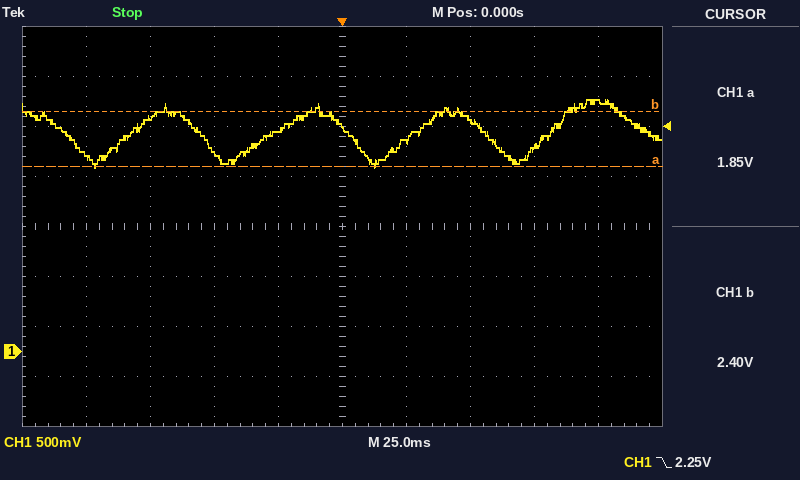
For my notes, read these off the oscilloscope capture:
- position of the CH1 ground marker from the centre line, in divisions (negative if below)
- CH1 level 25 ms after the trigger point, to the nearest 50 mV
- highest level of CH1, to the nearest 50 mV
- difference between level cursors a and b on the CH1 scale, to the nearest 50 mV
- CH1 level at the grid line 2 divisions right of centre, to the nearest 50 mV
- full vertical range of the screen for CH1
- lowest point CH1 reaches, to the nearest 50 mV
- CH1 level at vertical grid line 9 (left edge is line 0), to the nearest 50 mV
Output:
-2.5 div
2.10 V
2.50 V
550 mV
2.30 V
4 V
1.85 V
2.50 V
